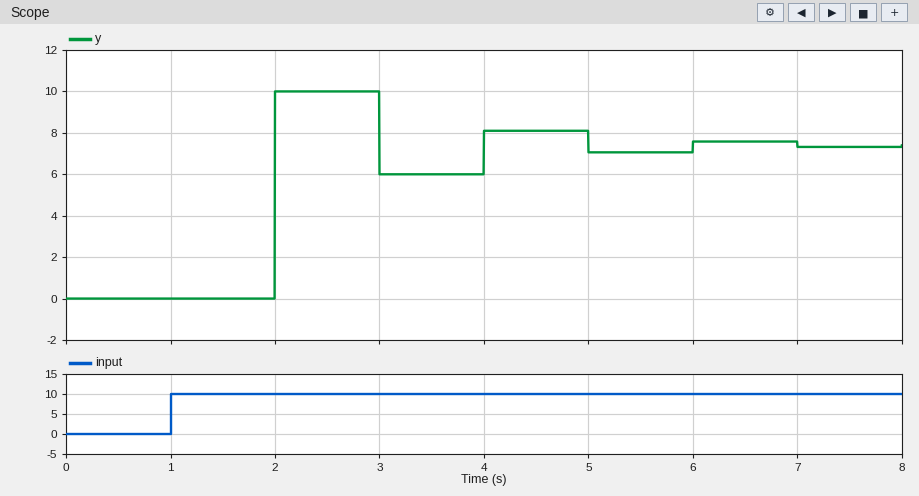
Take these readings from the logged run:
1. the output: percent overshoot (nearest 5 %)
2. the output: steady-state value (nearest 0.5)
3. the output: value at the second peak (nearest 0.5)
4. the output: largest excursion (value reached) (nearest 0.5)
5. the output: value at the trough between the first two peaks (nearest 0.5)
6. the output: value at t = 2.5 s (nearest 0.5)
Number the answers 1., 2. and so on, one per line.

1. 35 %
2. 7.5
3. 8.0
4. 10.0
5. 6.0
6. 10.0
